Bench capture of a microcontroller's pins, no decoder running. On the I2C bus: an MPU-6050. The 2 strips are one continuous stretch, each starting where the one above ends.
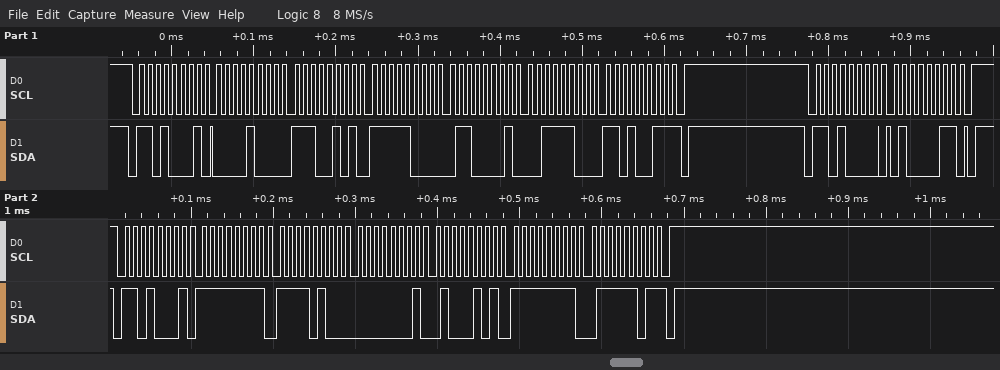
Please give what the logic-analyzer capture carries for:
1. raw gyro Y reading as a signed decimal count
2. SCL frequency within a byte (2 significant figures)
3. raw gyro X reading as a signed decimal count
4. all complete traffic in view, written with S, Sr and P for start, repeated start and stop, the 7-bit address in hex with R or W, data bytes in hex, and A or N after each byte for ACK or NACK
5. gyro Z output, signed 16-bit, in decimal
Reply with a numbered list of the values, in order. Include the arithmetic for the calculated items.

1. 0x0145 = 325
2. 100 kHz
3. 0xFFF4 = -12
4. S 68R A 08 A E5 A F8 A 61 A 3C A D3 N P S 68W A 43 A P S 68R A FF A F4 A 01 A 45 A FF A 7D N P
5. 0xFF7D = -131
